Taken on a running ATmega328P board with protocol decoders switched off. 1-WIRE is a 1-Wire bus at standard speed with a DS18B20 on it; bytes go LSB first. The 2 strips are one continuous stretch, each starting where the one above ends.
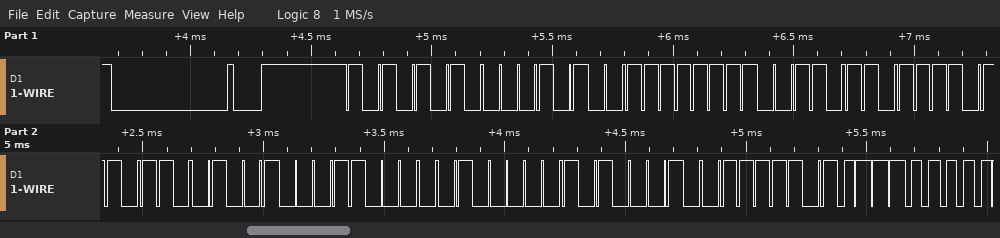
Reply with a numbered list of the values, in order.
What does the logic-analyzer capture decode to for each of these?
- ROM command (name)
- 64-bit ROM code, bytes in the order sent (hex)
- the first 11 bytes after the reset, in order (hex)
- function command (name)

1. Match ROM
2. 28 FF 6C 6F 93 18 04 45
3. 55 28 FF 6C 6F 93 18 04 45 BE 0E
4. Read Scratchpad
